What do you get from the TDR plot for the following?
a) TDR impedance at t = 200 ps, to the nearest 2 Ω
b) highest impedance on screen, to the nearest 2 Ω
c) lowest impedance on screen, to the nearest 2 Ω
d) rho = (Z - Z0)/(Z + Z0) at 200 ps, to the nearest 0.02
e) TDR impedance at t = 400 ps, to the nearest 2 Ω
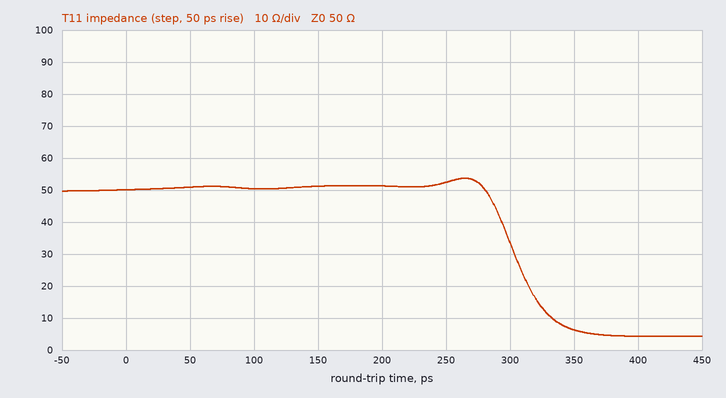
52 Ω
54 Ω
4 Ω
+0.02
4 Ω
